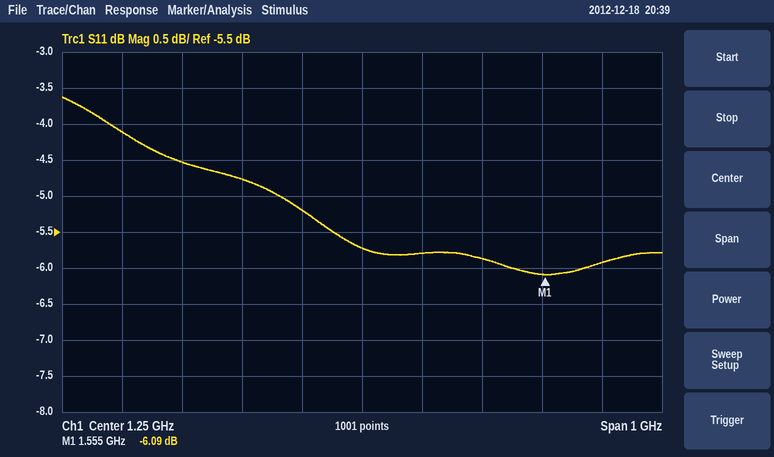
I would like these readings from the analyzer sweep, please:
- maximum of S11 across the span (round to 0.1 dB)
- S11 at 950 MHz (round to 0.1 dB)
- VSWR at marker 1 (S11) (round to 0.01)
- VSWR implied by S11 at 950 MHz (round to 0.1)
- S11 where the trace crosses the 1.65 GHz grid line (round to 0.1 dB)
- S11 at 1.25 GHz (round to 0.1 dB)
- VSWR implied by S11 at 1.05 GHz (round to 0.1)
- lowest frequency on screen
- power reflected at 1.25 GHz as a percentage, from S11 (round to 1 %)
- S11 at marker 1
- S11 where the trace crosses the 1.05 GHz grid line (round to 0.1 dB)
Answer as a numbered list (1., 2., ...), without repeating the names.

1. -3.6 dB
2. -4.5 dB
3. 2.97
4. 3.9
5. -5.9 dB
6. -5.7 dB
7. 3.7
8. 750 MHz
9. 27 %
10. -6.09 dB
11. -4.8 dB
